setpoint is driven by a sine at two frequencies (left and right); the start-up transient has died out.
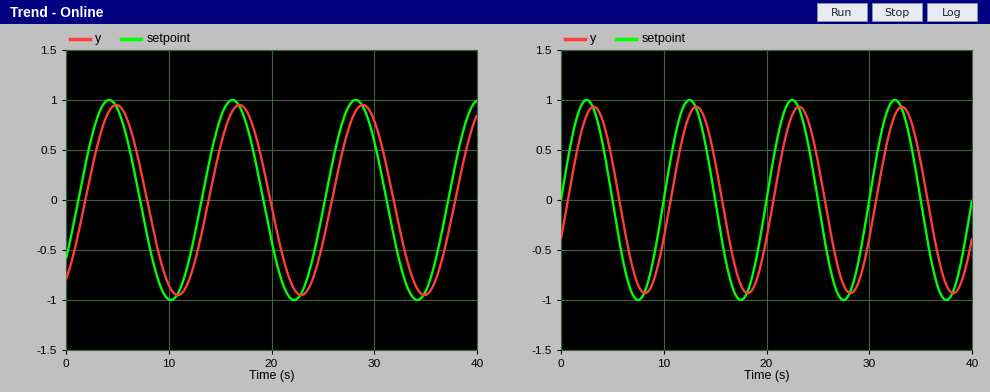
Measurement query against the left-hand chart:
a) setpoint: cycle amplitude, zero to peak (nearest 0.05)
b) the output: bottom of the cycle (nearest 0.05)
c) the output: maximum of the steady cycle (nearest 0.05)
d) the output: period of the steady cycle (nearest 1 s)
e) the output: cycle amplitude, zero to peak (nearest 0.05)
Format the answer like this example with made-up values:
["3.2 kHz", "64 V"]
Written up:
["1.00", "-0.95", "0.95", "12 s", "0.95"]
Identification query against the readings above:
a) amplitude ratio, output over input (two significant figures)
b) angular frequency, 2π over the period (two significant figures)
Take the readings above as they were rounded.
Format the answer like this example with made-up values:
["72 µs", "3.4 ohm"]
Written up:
["0.95", "0.52 rad/s"]
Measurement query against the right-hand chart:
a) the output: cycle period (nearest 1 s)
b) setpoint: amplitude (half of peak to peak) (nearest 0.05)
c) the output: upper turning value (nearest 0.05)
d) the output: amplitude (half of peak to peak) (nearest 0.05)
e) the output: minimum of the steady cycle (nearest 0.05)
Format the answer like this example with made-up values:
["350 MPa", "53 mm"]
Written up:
["10 s", "1.00", "0.95", "0.95", "-0.95"]
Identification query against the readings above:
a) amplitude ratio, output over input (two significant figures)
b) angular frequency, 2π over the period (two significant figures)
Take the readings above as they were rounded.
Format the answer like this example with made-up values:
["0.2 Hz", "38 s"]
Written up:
["0.95", "0.63 rad/s"]
